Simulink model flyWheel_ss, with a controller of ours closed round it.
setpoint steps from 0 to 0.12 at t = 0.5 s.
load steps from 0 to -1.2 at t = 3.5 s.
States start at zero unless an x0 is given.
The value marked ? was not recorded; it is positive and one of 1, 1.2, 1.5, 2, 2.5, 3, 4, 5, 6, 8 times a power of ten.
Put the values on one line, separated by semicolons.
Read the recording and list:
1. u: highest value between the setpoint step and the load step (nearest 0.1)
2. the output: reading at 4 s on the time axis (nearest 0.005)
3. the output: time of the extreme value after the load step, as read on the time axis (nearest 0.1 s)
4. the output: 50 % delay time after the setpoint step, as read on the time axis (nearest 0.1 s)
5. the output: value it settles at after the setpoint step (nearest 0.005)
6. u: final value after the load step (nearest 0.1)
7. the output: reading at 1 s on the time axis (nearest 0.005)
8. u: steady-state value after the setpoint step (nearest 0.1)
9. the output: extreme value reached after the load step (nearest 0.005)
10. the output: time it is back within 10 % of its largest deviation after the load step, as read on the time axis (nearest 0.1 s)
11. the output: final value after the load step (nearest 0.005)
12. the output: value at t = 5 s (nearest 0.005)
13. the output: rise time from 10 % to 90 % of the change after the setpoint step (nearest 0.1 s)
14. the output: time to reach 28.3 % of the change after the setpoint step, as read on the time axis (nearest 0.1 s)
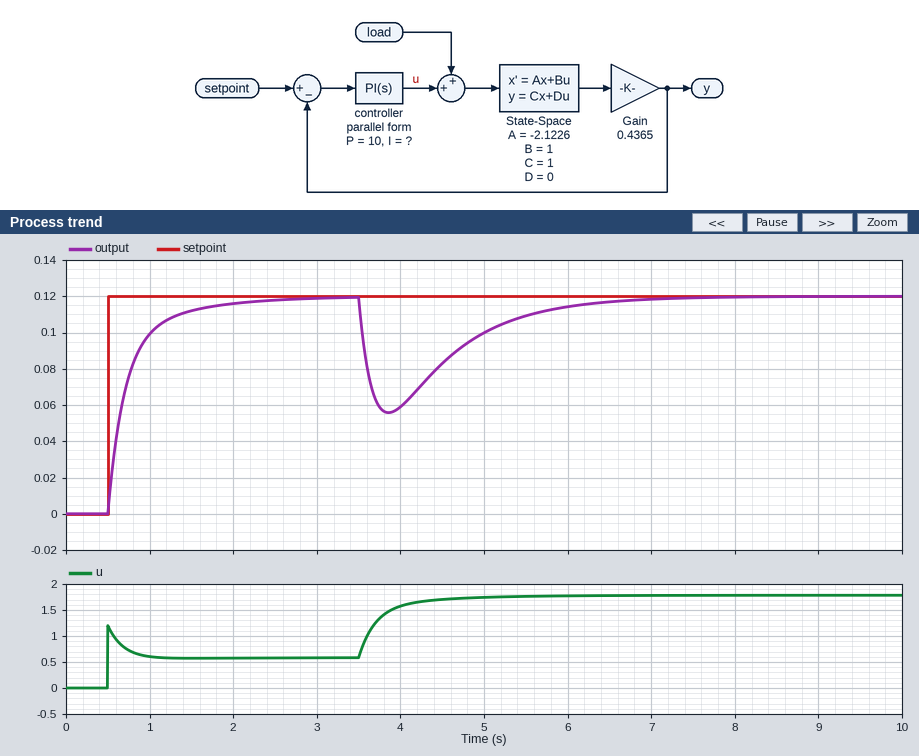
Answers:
1.2; 0.060; 3.9 s; 0.7 s; 0.120; 1.8; 0.100; 0.6; 0.055; 5.9 s; 0.120; 0.100; 0.7 s; 0.6 s
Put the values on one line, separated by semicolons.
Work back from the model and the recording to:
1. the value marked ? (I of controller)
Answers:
15
